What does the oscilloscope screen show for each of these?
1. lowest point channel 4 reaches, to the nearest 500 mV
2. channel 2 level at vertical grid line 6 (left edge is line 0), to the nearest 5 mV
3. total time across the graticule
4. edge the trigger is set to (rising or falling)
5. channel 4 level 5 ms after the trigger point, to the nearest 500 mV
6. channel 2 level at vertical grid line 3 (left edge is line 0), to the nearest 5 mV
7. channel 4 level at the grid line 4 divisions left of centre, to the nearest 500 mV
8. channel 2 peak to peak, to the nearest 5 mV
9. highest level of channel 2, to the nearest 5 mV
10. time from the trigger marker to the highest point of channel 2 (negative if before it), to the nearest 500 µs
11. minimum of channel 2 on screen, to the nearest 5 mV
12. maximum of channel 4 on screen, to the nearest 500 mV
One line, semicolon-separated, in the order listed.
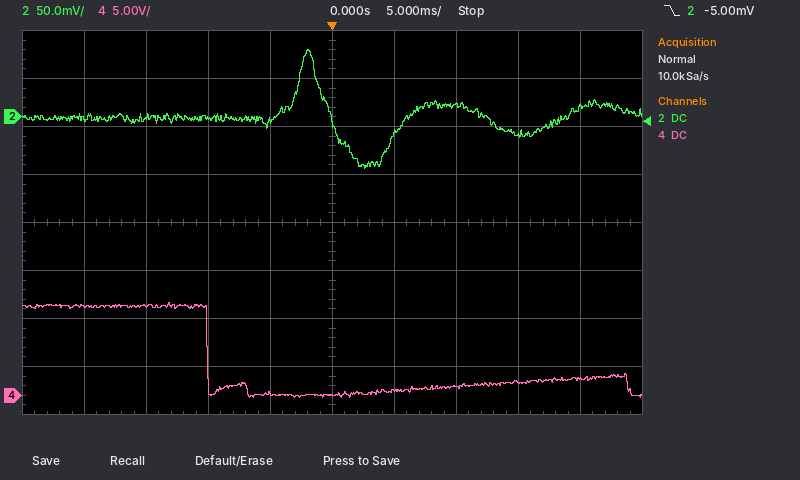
0.0 V; -20 mV; 50 ms; falling; 500 mV; 0 mV; 9.5 V; 125 mV; 70 mV; -2.0 ms; -55 mV; 9.5 V
